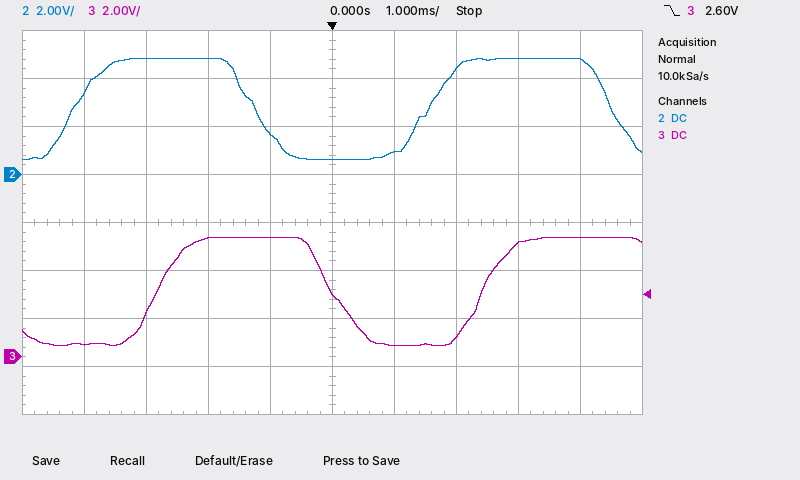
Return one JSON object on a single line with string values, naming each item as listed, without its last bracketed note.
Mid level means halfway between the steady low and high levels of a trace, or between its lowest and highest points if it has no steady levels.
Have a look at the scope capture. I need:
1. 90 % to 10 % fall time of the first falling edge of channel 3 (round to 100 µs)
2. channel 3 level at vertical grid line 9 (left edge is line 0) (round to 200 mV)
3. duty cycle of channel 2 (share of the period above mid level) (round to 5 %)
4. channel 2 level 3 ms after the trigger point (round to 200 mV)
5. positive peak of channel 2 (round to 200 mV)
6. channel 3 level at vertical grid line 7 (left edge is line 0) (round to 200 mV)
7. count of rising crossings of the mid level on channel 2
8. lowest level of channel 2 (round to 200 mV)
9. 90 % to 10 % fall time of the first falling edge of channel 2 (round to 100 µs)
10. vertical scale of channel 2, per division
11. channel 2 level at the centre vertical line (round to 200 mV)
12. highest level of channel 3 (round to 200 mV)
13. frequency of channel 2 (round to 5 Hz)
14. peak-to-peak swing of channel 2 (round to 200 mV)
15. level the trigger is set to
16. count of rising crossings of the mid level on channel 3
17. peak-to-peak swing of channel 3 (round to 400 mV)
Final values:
{"90 % to 10 % fall time of the first falling edge of channel 3": "900 µs", "channel 3 level at vertical grid line 9 (left edge is line 0)": "5.0 V", "duty cycle of channel 2 (share of the period above mid level)": "50 %", "channel 2 level 3 ms after the trigger point": "4.8 V", "positive peak of channel 2": "4.8 V", "channel 3 level at vertical grid line 7 (left edge is line 0)": "800 mV", "count of rising crossings of the mid level on channel 2": "2", "lowest level of channel 2": "600 mV", "90 % to 10 % fall time of the first falling edge of channel 2": "800 µs", "vertical scale of channel 2, per division": "2 V", "channel 2 level at the centre vertical line": "600 mV", "highest level of channel 3": "5.0 V", "frequency of channel 2": "175 Hz", "peak-to-peak swing of channel 2": "4.2 V", "level the trigger is set to": "2.60 V", "count of rising crossings of the mid level on channel 3": "2", "peak-to-peak swing of channel 3": "4.4 V"}
